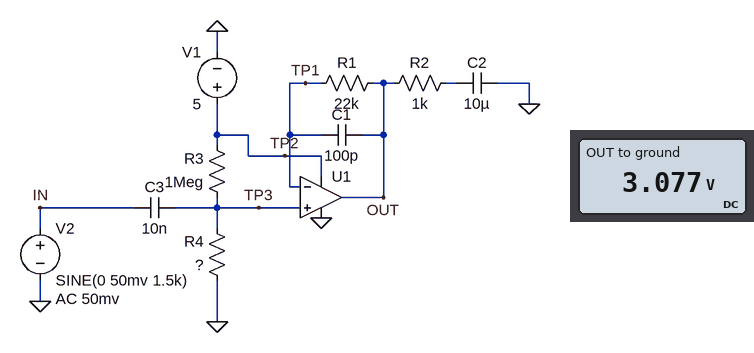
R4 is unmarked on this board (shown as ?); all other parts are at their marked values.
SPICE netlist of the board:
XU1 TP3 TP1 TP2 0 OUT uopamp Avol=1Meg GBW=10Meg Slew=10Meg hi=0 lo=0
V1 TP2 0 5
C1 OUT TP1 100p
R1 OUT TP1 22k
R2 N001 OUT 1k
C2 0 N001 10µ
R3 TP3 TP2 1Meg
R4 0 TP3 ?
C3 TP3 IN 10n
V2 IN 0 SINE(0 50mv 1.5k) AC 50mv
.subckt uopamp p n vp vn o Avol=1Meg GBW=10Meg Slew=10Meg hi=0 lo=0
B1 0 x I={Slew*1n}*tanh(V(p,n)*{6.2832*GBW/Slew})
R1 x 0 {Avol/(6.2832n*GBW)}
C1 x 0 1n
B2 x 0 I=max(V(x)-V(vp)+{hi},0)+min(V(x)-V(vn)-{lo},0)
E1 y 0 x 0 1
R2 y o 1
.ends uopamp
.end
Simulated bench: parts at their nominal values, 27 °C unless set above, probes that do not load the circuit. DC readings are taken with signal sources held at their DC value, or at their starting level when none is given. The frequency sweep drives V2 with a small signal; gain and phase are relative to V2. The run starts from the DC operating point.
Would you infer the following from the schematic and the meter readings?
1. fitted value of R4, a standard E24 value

1.6 MΩ
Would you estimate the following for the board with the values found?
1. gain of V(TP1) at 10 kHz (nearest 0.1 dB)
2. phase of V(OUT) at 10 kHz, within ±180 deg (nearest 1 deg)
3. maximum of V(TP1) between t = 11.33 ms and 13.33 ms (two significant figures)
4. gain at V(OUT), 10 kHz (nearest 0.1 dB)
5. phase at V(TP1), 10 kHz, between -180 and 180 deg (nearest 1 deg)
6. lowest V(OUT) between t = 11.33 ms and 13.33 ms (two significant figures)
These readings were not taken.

0 dB
0 deg
3.1 V
0 dB
0 deg
3.0 V
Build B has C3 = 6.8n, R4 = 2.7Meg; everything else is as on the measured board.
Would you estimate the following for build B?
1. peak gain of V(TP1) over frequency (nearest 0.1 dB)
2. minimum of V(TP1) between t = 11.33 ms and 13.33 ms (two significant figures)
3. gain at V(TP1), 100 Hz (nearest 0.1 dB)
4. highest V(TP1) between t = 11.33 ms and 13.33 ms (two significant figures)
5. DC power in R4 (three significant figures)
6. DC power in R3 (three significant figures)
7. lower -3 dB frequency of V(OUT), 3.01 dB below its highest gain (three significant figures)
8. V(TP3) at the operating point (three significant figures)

0 dB
3.6 V
-0.4 dB
3.7 V
4.93 µW
1.83 µW
32.1 Hz
3.65 V
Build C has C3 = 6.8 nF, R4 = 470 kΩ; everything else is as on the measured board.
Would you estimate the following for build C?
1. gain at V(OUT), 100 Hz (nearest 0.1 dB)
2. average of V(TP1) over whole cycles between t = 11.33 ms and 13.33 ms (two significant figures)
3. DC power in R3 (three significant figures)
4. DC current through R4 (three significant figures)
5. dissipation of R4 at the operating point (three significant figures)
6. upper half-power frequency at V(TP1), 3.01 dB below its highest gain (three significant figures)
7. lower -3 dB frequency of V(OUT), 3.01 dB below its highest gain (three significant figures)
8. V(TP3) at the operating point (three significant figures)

-1.9 dB
1.6 V
11.6 µW
3.40 µA
5.44 µW
9.99 MHz
73.2 Hz
1.60 V
